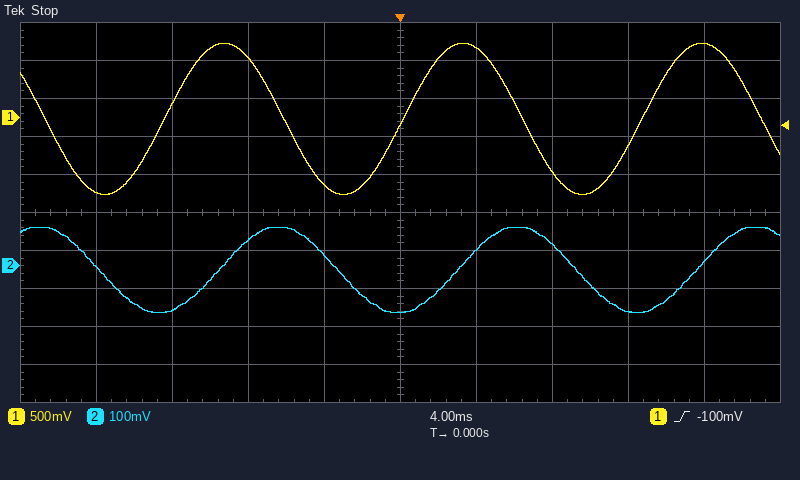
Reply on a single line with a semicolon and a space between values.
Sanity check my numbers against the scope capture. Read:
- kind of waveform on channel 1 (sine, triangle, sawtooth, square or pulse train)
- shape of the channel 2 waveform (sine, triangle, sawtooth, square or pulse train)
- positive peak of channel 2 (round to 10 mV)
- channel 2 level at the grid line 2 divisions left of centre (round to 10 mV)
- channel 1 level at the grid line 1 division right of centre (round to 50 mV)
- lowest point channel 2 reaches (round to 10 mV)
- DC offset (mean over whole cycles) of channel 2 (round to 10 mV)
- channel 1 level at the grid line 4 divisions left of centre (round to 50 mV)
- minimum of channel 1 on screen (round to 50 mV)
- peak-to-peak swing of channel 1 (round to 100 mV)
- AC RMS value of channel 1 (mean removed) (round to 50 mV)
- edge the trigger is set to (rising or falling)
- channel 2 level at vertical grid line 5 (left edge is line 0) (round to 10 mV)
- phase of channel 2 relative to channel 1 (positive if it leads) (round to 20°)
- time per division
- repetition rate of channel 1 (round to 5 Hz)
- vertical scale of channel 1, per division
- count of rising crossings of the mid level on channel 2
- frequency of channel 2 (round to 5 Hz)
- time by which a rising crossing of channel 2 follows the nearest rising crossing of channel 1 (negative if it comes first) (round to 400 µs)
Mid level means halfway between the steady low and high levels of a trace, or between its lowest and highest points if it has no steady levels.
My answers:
sine; sine; 100 mV; 70 mV; 900 mV; -120 mV; -10 mV; -1.00 V; -1.00 V; 2.00 V; 700 mV; rising; -120 mV; -80°; 4 ms; 80 Hz; 500 mV; 3; 80 Hz; +2.8 ms
